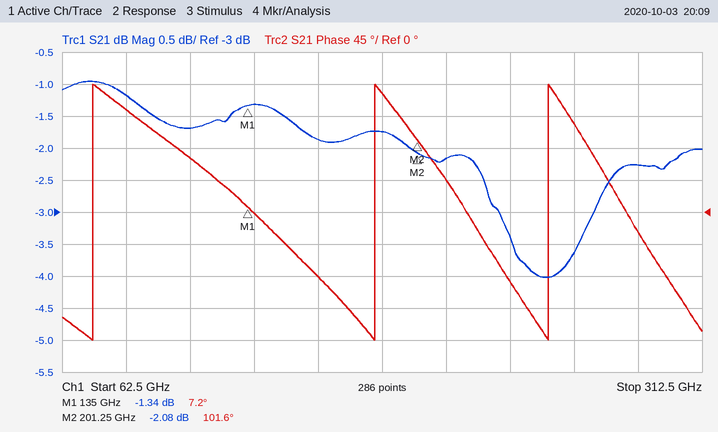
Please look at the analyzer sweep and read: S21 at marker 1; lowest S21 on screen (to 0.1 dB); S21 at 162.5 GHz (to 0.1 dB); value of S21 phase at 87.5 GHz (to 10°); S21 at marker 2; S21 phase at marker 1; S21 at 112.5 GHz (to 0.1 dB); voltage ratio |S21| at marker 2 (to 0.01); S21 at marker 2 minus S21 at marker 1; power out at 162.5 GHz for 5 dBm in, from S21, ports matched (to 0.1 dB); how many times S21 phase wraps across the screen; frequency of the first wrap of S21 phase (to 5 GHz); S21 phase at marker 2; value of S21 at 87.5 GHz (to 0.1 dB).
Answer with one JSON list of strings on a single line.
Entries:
["-1.34 dB", "-4.0 dB", "-1.9 dB", "140°", "-2.08 dB", "7.2°", "-1.7 dB", "0.79", "-0.74 dB", "3.1 dBm", "3", "75 GHz", "101.6°", "-1.2 dB"]
